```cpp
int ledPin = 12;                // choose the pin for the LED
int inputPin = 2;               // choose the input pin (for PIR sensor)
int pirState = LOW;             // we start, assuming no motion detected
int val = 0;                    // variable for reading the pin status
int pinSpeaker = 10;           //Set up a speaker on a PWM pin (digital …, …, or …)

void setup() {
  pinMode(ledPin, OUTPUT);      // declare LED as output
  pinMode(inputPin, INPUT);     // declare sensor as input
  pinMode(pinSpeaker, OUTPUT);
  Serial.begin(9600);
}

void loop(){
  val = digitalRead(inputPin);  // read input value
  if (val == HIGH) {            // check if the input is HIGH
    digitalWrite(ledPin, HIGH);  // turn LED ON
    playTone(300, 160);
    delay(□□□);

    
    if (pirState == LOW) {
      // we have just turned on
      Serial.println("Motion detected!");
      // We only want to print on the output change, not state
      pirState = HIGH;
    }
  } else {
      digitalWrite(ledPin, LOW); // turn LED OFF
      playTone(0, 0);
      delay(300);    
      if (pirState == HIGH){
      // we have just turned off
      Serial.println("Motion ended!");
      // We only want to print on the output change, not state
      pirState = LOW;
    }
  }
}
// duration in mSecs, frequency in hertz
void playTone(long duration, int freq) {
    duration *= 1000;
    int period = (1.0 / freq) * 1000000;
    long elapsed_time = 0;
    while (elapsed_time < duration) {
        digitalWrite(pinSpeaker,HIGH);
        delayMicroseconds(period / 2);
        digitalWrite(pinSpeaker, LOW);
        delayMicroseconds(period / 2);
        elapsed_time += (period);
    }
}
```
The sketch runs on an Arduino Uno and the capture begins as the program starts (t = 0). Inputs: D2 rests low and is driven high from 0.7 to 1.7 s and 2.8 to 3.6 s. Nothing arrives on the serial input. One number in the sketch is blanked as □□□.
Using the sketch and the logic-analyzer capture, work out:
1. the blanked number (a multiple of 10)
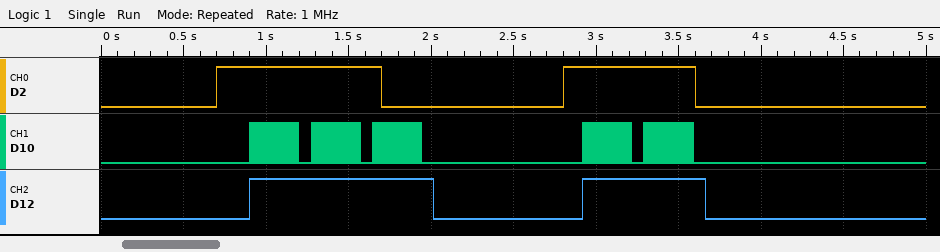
70
